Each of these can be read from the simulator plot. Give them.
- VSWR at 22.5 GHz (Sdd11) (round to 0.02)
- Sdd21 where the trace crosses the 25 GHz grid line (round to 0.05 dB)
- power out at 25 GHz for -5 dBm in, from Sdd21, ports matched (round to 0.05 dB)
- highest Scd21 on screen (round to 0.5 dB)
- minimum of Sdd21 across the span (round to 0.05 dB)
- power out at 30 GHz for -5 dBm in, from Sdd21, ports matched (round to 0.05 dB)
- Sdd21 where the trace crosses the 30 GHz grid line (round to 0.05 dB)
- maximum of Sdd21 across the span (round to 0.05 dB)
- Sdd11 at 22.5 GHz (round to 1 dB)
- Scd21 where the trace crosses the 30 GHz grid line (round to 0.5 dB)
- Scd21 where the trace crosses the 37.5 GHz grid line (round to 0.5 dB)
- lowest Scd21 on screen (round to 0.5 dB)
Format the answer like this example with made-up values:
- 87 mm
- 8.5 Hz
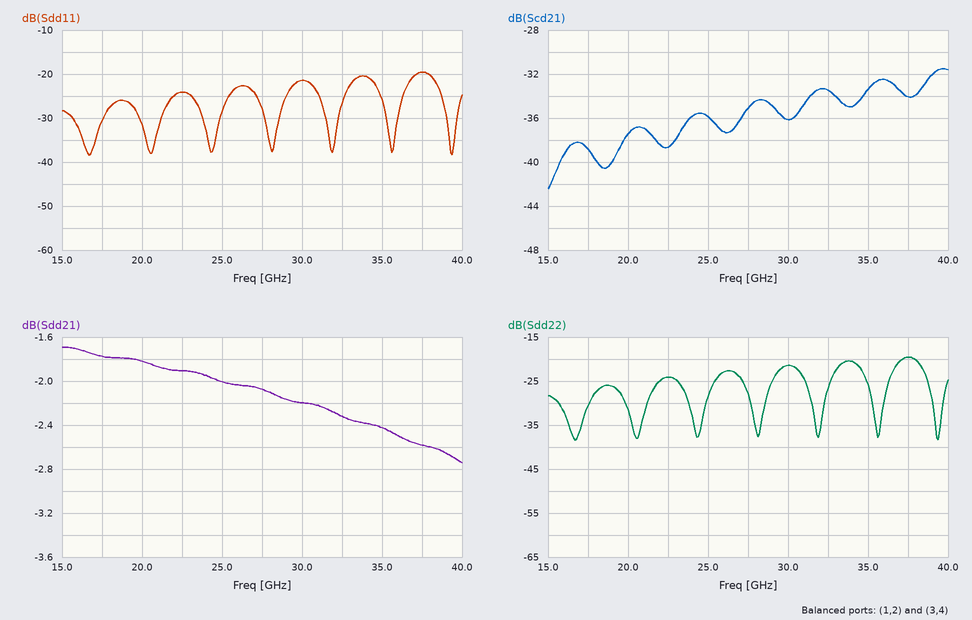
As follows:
- 1.14
- -2.00 dB
- -7.00 dBm
- -31.5 dB
- -2.75 dB
- -7.20 dBm
- -2.20 dB
- -1.70 dB
- -24 dB
- -36.0 dB
- -34.0 dB
- -42.5 dB
